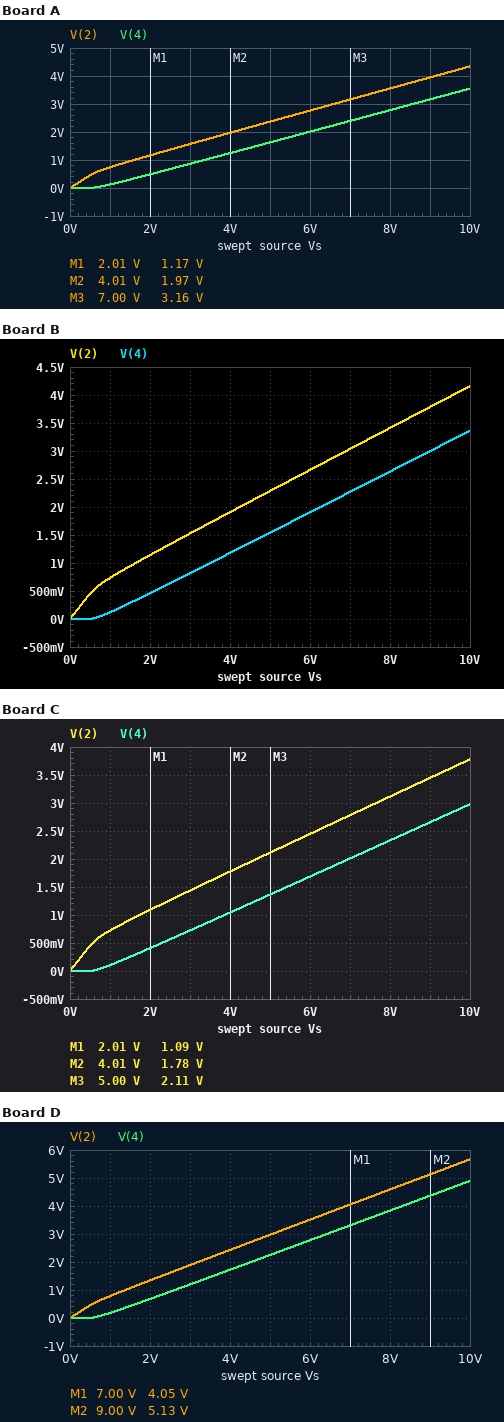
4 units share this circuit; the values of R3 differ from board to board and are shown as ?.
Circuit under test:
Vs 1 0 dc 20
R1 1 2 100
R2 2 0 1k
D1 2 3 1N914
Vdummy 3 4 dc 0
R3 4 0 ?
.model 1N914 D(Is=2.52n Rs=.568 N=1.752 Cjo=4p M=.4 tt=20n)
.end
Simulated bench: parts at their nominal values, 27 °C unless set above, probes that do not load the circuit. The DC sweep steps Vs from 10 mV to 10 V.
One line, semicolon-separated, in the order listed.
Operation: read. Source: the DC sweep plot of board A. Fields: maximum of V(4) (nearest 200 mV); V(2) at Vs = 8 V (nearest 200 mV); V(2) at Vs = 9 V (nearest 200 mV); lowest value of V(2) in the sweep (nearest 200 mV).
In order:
3.6 V; 3.6 V; 4.0 V; 0 V
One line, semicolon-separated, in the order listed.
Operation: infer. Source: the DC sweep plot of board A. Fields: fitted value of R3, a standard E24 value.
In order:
68 Ω
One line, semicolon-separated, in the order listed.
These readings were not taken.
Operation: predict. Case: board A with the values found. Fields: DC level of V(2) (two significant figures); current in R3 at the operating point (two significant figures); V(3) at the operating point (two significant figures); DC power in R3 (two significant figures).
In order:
8.3 V; 110 mA; 7.4 V; 810 mW
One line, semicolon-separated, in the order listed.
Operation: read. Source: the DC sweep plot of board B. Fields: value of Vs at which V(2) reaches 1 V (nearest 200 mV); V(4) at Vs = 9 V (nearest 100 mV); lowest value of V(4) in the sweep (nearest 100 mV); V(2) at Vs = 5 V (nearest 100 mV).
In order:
1.6 V; 3.0 V; 0 V; 2.3 V
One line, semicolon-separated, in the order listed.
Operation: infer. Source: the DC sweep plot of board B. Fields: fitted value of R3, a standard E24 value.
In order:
62 Ω
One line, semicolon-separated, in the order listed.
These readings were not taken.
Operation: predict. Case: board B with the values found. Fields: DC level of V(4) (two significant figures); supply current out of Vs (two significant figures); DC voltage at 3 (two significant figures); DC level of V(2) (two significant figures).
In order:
7.0 V; 120 mA; 7.0 V; 7.9 V
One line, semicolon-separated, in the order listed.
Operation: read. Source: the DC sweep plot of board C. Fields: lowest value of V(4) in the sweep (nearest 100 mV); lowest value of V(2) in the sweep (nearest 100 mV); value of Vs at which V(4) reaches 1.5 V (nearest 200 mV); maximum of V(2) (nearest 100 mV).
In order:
0 V; 0 V; 5.4 V; 3.8 V
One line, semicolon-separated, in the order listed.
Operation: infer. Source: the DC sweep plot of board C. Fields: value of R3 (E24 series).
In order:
51 Ω
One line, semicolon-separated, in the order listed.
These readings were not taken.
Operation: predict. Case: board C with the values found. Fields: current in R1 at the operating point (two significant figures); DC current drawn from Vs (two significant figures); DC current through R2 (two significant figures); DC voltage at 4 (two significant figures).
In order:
130 mA; 130 mA; 7.1 mA; 6.2 V
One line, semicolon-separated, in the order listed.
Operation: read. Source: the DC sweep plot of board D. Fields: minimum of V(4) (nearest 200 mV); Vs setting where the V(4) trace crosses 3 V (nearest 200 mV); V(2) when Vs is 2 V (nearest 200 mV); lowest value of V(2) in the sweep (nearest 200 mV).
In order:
0 V; 6.4 V; 1.4 V; 0 V
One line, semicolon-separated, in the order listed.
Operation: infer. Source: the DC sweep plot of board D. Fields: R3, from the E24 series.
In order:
130 Ω
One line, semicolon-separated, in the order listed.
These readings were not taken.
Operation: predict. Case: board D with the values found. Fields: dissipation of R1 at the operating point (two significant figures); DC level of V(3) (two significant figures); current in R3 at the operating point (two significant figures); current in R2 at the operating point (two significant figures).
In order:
800 mW; 10 V; 79 mA; 11 mA
